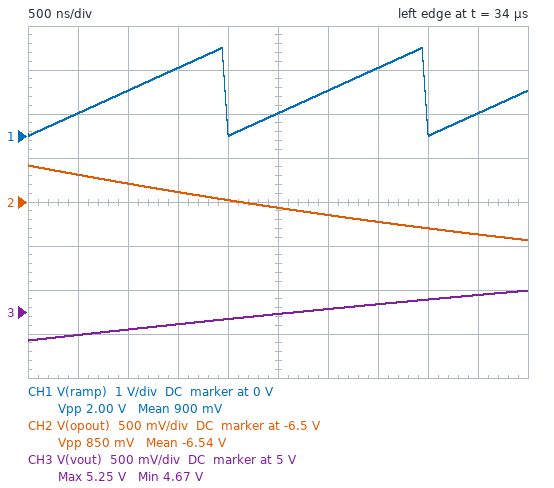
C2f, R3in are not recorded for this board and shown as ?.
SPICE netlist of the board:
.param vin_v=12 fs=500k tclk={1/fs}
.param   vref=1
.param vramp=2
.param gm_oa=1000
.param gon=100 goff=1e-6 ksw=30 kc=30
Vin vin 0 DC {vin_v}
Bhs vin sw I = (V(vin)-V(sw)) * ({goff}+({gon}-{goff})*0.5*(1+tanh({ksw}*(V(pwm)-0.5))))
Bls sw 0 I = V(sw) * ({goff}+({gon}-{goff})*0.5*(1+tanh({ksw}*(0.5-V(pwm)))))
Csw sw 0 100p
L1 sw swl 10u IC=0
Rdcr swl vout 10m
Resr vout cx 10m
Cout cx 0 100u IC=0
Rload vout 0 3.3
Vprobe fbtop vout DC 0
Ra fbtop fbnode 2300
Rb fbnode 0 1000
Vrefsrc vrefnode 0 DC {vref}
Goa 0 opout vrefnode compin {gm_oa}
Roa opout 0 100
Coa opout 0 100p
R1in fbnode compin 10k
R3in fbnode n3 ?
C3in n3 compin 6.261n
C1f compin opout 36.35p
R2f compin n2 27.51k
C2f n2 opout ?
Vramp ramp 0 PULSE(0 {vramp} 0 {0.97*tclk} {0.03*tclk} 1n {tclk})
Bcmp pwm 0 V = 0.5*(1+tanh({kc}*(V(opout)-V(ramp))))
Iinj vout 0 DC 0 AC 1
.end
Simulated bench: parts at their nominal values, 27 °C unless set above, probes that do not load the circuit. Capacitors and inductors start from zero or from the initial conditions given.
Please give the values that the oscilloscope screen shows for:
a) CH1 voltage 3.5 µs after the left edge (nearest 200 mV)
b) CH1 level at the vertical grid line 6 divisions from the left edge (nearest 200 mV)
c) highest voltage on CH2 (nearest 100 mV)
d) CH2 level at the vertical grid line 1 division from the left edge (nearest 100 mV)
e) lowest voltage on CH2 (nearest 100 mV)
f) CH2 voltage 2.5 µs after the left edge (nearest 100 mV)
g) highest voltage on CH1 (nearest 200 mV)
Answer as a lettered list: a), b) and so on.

a) 1.6 V
b) 1.0 V
c) -6.1 V
d) -6.2 V
e) -6.9 V
f) -6.6 V
g) 2.0 V
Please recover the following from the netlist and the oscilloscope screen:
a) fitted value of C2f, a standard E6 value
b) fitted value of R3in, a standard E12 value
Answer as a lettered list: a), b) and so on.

a) 1 nF
b) 220 Ω
